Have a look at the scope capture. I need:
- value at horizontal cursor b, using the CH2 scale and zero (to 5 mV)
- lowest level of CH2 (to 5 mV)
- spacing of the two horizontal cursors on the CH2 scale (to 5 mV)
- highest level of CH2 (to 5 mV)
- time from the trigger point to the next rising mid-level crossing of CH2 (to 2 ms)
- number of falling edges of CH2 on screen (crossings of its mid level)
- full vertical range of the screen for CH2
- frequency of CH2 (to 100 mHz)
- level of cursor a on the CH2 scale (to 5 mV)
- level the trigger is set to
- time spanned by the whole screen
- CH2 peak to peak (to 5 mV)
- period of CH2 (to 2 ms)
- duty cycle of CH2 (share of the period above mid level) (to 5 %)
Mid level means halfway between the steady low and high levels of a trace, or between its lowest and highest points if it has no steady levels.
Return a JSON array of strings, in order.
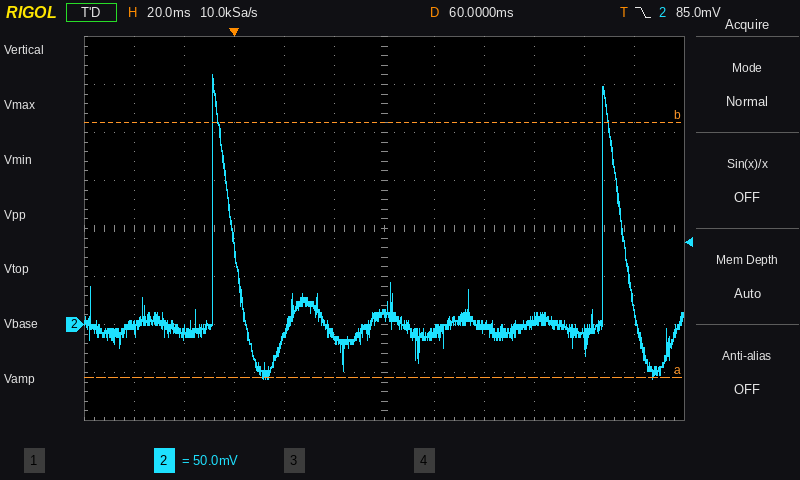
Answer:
["210 mV", "-55 mV", "265 mV", "260 mV", "148 ms", "2", "400 mV", "6.4 Hz", "-55 mV", "85.0 mV", "240 ms", "315 mV", "156 ms", "5 %"]
